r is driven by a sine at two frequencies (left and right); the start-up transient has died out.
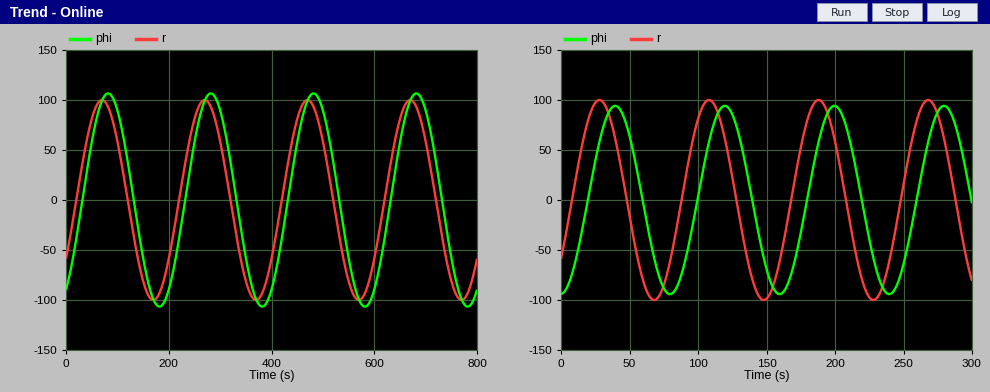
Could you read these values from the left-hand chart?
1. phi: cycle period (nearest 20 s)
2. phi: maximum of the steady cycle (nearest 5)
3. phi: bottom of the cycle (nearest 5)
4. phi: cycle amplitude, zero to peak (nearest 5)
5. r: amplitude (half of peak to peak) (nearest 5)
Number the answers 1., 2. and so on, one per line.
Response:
1. 200 s
2. 105
3. -105
4. 105
5. 100
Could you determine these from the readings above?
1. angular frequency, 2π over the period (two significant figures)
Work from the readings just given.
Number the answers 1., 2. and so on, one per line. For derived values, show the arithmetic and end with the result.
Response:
1. 2π / 200 = 0.031 rad/s
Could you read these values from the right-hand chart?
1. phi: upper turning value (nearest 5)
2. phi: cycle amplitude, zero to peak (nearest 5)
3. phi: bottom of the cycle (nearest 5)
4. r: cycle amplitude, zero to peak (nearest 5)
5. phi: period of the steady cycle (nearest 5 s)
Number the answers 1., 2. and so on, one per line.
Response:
1. 95
2. 95
3. -95
4. 100
5. 80 s
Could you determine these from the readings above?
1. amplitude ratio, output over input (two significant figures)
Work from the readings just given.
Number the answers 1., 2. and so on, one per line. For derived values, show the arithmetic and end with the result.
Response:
1. 95 / 100 = 0.95
